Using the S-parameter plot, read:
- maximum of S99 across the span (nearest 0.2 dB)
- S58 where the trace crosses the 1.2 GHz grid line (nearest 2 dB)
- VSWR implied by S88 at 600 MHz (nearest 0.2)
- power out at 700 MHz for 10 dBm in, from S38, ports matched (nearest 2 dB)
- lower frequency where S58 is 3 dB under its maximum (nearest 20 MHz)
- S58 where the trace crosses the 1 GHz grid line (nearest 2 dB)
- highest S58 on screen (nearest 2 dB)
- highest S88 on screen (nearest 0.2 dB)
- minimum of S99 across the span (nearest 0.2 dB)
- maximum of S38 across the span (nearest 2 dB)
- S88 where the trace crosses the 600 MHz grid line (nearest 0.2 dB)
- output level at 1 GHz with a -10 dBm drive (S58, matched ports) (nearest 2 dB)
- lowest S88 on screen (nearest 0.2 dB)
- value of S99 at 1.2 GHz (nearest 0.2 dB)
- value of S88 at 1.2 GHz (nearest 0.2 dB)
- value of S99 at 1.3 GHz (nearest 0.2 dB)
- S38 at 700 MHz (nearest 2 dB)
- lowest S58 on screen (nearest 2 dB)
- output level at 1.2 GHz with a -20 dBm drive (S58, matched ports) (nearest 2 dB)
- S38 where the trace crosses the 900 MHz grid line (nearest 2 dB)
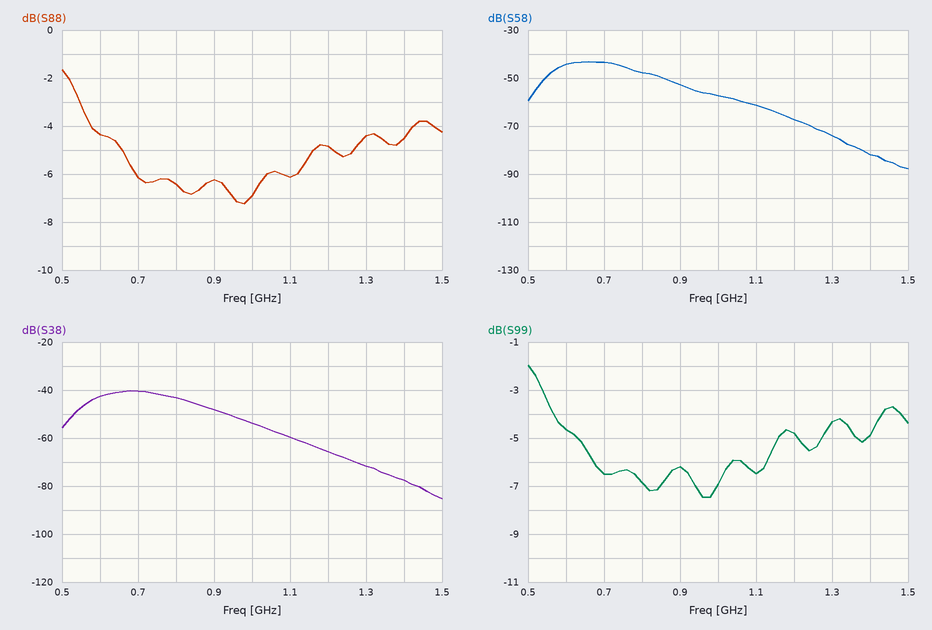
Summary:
-2.0 dB
-68 dB
4.0
-30 dBm
580 MHz
-58 dB
-44 dB
-1.6 dB
-7.4 dB
-40 dB
-4.4 dB
-68 dBm
-7.2 dB
-4.8 dB
-4.8 dB
-4.4 dB
-40 dB
-88 dB
-88 dBm
-48 dB
